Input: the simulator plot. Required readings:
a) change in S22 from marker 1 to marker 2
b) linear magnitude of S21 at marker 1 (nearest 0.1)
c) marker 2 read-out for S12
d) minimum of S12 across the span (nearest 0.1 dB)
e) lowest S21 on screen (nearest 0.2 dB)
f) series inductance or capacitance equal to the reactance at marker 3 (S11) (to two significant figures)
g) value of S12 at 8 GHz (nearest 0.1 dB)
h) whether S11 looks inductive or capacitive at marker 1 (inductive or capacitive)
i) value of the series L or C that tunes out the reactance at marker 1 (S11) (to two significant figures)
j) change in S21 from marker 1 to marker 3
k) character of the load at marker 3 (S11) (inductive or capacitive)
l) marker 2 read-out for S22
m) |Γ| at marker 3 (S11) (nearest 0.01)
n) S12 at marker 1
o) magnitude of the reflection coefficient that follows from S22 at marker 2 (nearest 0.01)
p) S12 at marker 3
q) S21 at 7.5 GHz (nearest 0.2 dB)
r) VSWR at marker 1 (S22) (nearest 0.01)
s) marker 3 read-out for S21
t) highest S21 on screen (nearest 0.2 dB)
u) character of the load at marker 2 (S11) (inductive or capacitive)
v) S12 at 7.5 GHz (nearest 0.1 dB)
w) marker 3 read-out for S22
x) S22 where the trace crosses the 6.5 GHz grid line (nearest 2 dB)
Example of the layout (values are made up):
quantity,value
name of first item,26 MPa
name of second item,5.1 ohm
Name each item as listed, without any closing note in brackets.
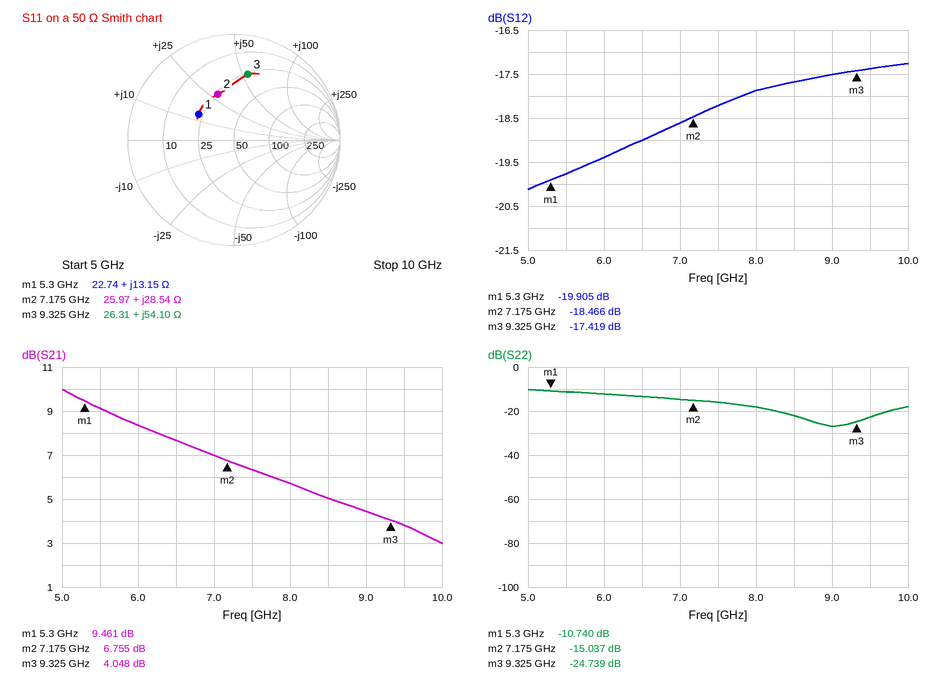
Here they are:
quantity,value
change in S22 from marker 1 to marker 2,-4.297 dB
linear magnitude of S21 at marker 1,3.0
marker 2 read-out for S12,-18.466 dB
minimum of S12 across the span,-20.1 dB
lowest S21 on screen,3.0 dB
series inductance or capacitance equal to the reactance at marker 3 (S11),920 pH
value of S12 at 8 GHz,-17.9 dB
whether S11 looks inductive or capacitive at marker 1,inductive
value of the series L or C that tunes out the reactance at marker 1 (S11),2.3 pF
change in S21 from marker 1 to marker 3,-5.413 dB
character of the load at marker 3 (S11),inductive
marker 2 read-out for S22,-15.037 dB
|Γ| at marker 3 (S11),0.63
S12 at marker 1,-19.905 dB
magnitude of the reflection coefficient that follows from S22 at marker 2,0.18
S12 at marker 3,-17.419 dB
S21 at 7.5 GHz,6.4 dB
VSWR at marker 1 (S22),1.82
marker 3 read-out for S21,4.048 dB
highest S21 on screen,10.0 dB
character of the load at marker 2 (S11),inductive
S12 at 7.5 GHz,-18.2 dB
marker 3 read-out for S22,-24.739 dB
S22 where the trace crosses the 6.5 GHz grid line,-14 dB
